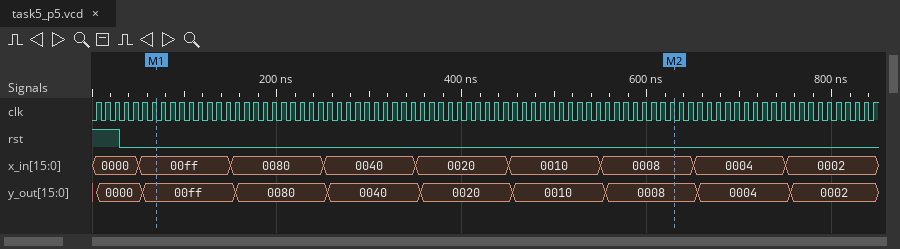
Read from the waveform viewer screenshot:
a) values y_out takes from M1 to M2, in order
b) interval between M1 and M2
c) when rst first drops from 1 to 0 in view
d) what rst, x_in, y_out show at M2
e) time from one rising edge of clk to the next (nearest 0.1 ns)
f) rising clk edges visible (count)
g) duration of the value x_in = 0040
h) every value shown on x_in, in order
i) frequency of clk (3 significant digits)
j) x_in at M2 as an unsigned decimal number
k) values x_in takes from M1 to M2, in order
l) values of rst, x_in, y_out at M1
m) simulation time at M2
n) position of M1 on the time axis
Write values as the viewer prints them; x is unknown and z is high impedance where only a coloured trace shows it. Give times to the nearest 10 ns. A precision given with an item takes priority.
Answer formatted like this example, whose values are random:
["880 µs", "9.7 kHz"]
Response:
["00ff, 0080, 0040, 0020, 0010, 0008", "560 ns", "30 ns", "rst=0, x_in=0008, y_out=0008", "10 ns", "85", "100 ns", "0000, 00ff, 0080, 0040, 0020, 0010, 0008, 0004, 0002", "100 MHz", "8", "00ff, 0080, 0040, 0020, 0010, 0008", "rst=0, x_in=00ff, y_out=00ff", "630 ns", "70 ns"]
